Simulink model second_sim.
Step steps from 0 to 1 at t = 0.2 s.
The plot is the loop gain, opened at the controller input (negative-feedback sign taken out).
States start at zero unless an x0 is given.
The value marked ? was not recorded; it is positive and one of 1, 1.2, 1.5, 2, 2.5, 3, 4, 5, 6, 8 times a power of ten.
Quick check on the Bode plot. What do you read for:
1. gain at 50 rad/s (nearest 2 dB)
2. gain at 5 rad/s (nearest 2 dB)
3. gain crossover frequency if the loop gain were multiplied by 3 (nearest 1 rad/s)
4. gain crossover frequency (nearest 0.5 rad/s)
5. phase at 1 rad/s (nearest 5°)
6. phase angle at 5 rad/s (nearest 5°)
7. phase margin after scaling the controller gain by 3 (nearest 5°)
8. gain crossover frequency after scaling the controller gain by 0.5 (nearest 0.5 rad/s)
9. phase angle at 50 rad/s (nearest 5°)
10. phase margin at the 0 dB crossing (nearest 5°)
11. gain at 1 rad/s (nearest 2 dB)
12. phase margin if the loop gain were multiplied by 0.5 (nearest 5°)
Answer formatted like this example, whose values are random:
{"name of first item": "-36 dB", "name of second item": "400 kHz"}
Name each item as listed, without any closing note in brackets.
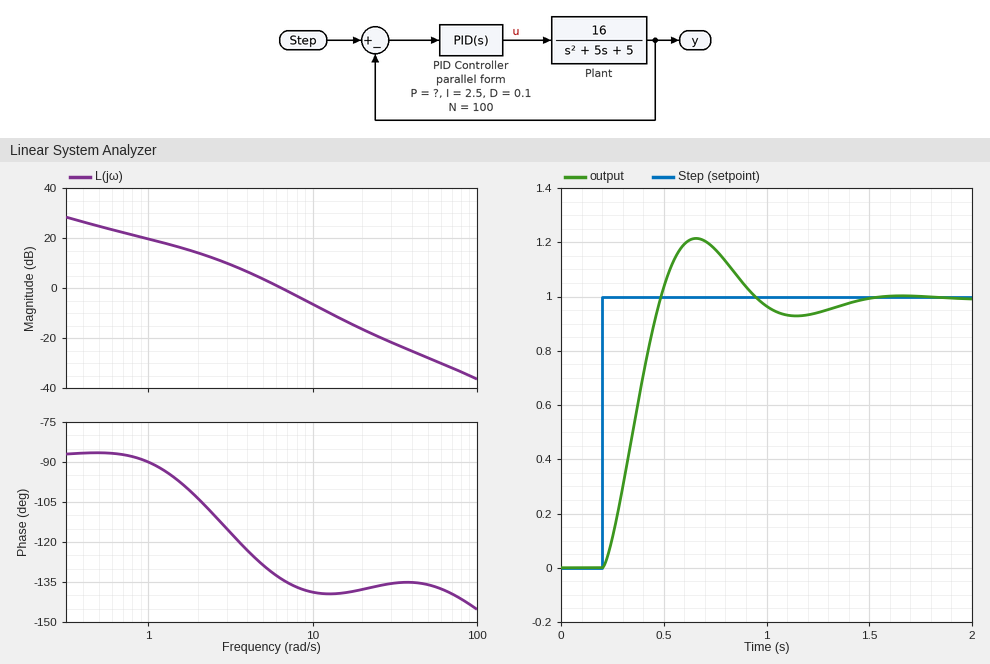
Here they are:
{"gain at 50 rad/s": "-28 dB", "gain at 5 rad/s": "4 dB", "gain crossover frequency if the loop gain were multiplied by 3": "12 rad/s", "gain crossover frequency": "6.5 rad/s", "phase at 1 rad/s": "-90°", "phase angle at 5 rad/s": "-130°", "phase margin after scaling the controller gain by 3": "40°", "gain crossover frequency after scaling the controller gain by 0.5": "4.0 rad/s", "phase angle at 50 rad/s": "-135°", "phase margin at the 0 dB crossing": "45°", "gain at 1 rad/s": "20 dB", "phase margin if the loop gain were multiplied by 0.5": "55°"}
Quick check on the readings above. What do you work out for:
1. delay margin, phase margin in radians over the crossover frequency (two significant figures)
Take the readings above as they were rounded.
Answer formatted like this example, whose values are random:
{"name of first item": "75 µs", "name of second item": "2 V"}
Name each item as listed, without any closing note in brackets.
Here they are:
{"delay margin, phase margin in radians over the crossover frequency": "0.12 s"}
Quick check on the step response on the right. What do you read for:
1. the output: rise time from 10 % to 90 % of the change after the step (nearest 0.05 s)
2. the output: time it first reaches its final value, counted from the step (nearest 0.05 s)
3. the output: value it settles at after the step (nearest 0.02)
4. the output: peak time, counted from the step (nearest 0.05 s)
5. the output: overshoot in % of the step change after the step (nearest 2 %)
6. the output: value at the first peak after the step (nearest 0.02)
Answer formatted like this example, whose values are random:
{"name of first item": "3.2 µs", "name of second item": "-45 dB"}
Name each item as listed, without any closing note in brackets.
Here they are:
{"the output: rise time from 10 % to 90 % of the change after the step": "0.20 s", "the output: time it first reaches its final value, counted from the step": "0.30 s", "the output: value it settles at after the step": "1.00", "the output: peak time, counted from the step": "0.45 s", "the output: overshoot in % of the step change after the step": "22 %", "the output: value at the first peak after the step": "1.22"}
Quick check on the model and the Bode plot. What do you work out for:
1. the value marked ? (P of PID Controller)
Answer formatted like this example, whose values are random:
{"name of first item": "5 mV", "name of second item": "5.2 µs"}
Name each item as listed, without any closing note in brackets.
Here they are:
{"the value marked ?": "3"}
